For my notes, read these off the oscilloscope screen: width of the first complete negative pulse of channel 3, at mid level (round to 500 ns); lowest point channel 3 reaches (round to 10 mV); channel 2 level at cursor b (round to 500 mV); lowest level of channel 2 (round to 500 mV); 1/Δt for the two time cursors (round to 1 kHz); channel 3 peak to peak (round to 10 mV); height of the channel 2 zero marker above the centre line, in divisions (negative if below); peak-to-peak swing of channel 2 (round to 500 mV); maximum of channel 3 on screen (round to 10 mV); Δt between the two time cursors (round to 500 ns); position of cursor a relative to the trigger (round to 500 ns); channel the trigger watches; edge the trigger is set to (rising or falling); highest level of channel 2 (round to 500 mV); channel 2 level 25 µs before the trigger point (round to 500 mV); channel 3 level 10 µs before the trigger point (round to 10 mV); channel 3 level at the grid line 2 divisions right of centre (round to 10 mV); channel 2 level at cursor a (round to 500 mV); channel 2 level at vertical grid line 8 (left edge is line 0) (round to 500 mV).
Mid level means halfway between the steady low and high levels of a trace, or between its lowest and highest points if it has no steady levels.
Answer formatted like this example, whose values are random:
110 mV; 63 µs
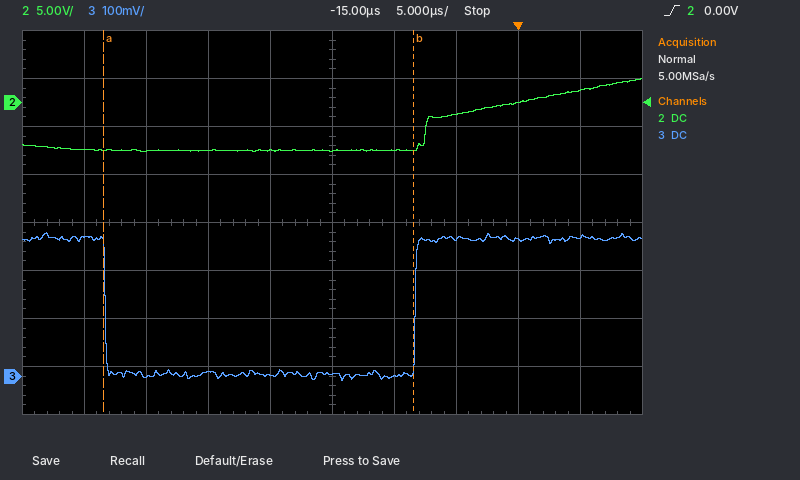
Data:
25.0 µs; -10 mV; -5.0 V; -5.0 V; 40 kHz; 310 mV; +2.5 div; 7.5 V; 300 mV; 25.0 µs; -33.5 µs; channel 2; rising; 2.5 V; -5.0 V; 0 mV; 290 mV; -5.0 V; 0.0 V
